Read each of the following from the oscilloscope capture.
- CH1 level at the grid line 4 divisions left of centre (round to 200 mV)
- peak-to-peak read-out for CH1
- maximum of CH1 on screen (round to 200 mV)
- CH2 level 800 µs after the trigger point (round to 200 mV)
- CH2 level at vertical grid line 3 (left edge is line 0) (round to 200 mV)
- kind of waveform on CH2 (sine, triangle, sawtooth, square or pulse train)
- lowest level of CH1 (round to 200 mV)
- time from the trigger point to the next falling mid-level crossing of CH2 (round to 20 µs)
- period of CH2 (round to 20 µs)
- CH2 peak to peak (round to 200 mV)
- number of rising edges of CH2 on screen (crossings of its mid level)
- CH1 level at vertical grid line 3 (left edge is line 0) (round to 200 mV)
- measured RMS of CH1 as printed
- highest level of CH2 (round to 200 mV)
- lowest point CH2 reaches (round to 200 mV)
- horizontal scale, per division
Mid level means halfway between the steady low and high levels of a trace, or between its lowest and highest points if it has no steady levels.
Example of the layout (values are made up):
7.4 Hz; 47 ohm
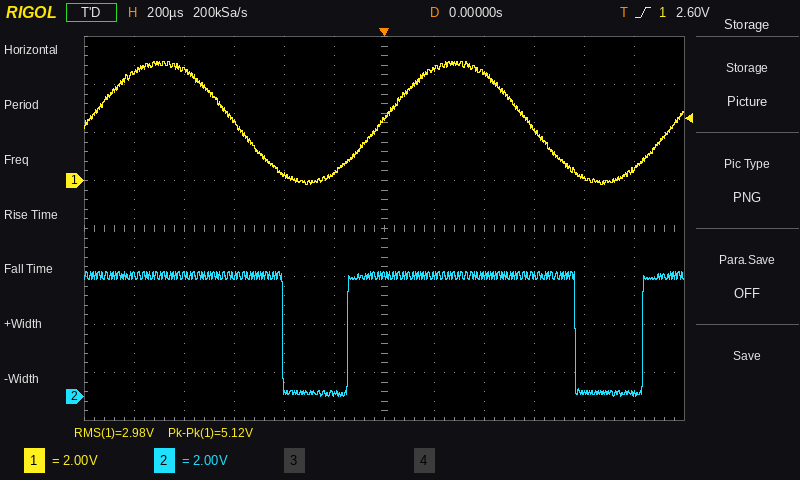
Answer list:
4.6 V; 5.12 V; 5.0 V; 200 mV; 5.0 V; pulse train; -200 mV; 760 µs; 1.18 ms; 5.2 V; 2; 2.4 V; 2.98 V; 5.2 V; 0.0 V; 200 µs
